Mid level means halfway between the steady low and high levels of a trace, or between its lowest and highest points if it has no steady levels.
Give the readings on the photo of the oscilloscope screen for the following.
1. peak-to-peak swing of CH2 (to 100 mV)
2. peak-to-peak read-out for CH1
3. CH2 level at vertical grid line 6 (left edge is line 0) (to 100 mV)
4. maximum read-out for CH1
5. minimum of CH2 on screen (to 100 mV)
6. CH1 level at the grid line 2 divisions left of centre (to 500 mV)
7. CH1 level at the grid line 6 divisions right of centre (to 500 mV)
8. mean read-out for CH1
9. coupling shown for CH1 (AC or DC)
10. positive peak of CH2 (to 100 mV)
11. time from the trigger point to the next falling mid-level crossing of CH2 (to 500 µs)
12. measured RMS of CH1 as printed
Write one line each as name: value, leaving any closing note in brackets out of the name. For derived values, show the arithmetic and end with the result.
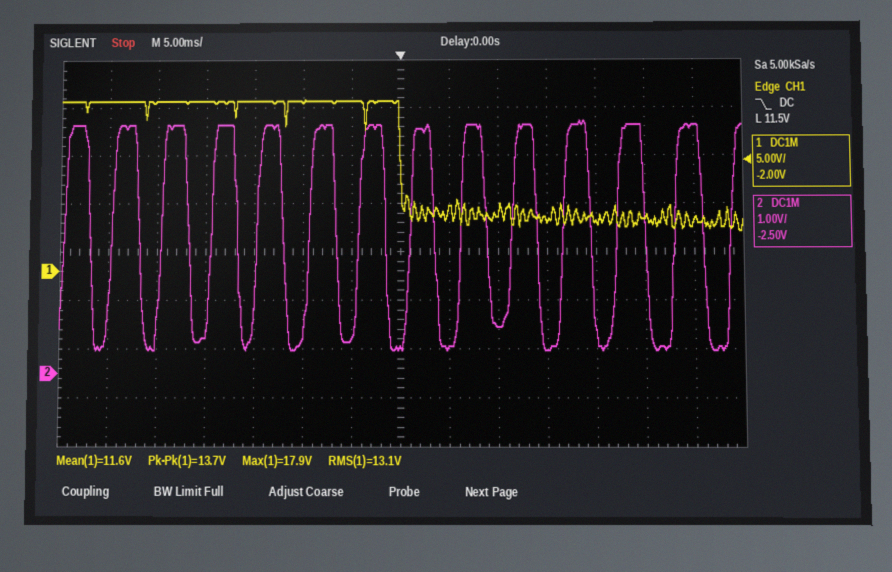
peak-to-peak swing of CH2: 5.2 V − (500 mV) = 4.7 V
peak-to-peak read-out for CH1: 13.7 V
CH2 level at vertical grid line 6 (left edge is line 0): 700 mV
maximum read-out for CH1: 17.9 V
minimum of CH2 on screen: 500 mV
CH1 level at the grid line 2 divisions left of centre: 17.5 V
CH1 level at the grid line 6 divisions right of centre: 5.0 V
mean read-out for CH1: 11.6 V
coupling shown for CH1: DC
positive peak of CH2: 5.2 V
time from the trigger point to the next falling mid-level crossing of CH2: 3.5 ms
measured RMS of CH1 as printed: 13.1 V
